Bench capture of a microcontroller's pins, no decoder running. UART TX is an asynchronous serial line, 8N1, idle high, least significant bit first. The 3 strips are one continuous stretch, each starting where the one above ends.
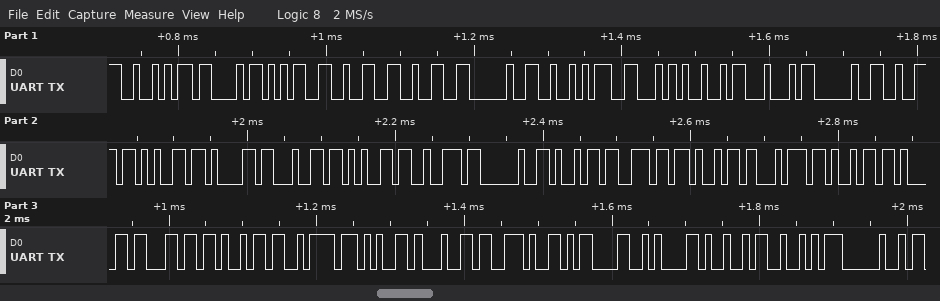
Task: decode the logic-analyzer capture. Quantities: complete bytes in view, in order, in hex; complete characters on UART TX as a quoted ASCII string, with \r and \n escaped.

0x52 0x43 0x35 0x32 0x32 0x20 0x52 0x46 0x49 0x44 0x20 0x72 0x65 0x61 0x64 0x65 0x72 0x20 0x69 0x6E 0x69 0x74 0x69 0x61 0x6C 0x69 0x7A 0x65 0x64 0x2E 0x0D 0x0A 0x49 0x52 0x20
"RC522 RFID reader initialized.\r\nIR "
